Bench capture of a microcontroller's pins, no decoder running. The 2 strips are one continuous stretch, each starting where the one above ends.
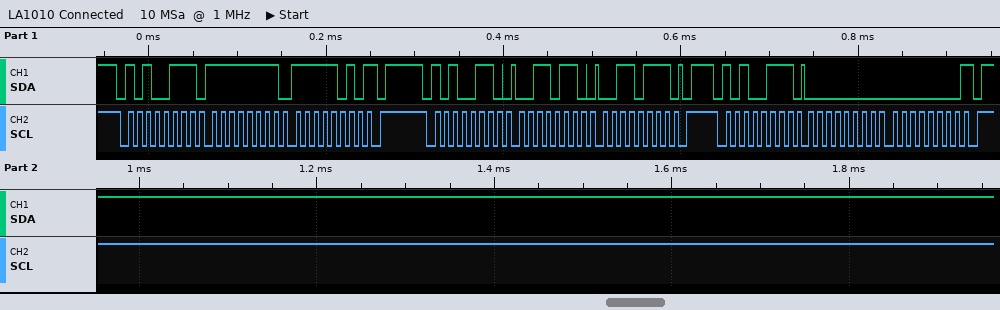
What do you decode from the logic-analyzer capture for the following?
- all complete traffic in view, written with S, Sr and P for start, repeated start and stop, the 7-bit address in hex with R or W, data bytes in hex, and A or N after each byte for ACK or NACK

S 53R A FF A FA N P S 53W A 36 A 37 A P S 53R A 00 A 00 N P
